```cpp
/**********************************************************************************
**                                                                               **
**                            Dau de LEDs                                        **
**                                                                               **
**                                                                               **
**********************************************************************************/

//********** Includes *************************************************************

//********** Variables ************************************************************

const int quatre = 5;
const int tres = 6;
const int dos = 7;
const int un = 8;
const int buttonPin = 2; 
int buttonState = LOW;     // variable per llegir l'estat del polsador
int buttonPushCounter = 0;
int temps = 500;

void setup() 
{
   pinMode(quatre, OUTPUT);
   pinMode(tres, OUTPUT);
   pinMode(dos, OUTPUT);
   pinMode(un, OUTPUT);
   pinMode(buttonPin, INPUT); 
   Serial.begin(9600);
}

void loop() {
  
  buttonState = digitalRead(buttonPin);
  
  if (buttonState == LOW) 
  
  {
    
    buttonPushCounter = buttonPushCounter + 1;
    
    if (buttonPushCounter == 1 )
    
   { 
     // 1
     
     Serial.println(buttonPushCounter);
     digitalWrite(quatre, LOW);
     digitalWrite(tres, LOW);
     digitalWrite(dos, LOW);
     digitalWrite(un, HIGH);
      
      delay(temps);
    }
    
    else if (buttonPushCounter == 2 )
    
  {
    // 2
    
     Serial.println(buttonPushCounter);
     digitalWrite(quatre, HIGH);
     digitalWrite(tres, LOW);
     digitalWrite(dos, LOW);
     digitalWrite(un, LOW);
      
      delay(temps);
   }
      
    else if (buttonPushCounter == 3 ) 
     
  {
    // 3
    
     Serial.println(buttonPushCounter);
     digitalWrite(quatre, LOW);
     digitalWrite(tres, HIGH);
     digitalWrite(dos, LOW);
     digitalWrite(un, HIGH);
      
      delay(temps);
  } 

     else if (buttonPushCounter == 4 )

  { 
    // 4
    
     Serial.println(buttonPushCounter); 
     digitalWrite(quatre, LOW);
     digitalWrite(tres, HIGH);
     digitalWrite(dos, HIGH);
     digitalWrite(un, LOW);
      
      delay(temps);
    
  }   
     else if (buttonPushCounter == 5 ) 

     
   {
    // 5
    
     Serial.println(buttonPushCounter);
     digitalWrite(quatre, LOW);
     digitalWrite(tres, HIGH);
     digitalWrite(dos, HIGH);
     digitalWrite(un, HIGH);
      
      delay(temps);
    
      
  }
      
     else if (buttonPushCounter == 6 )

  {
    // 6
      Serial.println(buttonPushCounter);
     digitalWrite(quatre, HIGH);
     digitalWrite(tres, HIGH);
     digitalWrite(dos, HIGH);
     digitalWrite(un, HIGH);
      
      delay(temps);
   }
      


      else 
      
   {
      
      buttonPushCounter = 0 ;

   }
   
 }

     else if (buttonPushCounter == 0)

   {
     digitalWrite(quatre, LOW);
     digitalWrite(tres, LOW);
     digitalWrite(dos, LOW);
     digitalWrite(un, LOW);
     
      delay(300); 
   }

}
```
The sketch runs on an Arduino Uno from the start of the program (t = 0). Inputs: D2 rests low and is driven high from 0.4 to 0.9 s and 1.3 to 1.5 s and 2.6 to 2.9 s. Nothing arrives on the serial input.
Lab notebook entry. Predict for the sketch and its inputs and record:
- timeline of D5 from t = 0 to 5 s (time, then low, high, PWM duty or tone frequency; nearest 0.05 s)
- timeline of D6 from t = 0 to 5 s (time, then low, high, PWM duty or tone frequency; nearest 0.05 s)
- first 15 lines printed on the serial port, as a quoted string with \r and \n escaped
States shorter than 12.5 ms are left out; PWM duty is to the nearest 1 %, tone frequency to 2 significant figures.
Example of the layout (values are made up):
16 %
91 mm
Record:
0 s low; 0.9 s high; 1.5 s low; 3 s high; 3.5 s low; 4 s high; 4.5 s low
0 s low; 1.5 s high; 3.5 s low; 4.5 s high
"1\r\n2\r\n3\r\n4\r\n5\r\n6\r\n1\r\n2\r\n3\r\n4\r\n5\r\n6\r\n1\r\n2\r\n3\r\n"
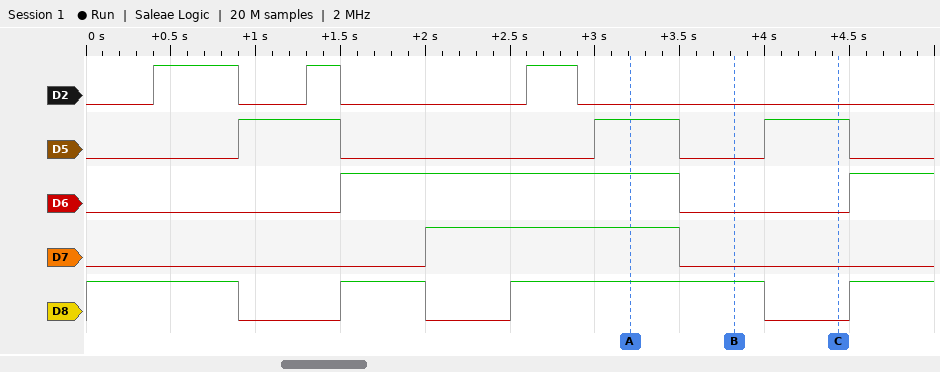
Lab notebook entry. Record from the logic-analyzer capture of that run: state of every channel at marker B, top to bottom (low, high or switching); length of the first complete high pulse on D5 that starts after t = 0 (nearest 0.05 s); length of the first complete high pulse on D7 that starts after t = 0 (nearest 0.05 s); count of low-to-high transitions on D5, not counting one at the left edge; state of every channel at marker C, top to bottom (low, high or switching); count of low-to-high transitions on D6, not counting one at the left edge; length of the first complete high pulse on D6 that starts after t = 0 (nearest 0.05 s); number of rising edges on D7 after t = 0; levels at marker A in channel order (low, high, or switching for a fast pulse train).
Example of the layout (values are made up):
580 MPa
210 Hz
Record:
D2 low, D5 low, D6 low, D7 low, D8 high
0.60 s
1.50 s
3
D2 low, D5 high, D6 low, D7 low, D8 low
2
2.00 s
1
D2 low, D5 high, D6 high, D7 high, D8 high
